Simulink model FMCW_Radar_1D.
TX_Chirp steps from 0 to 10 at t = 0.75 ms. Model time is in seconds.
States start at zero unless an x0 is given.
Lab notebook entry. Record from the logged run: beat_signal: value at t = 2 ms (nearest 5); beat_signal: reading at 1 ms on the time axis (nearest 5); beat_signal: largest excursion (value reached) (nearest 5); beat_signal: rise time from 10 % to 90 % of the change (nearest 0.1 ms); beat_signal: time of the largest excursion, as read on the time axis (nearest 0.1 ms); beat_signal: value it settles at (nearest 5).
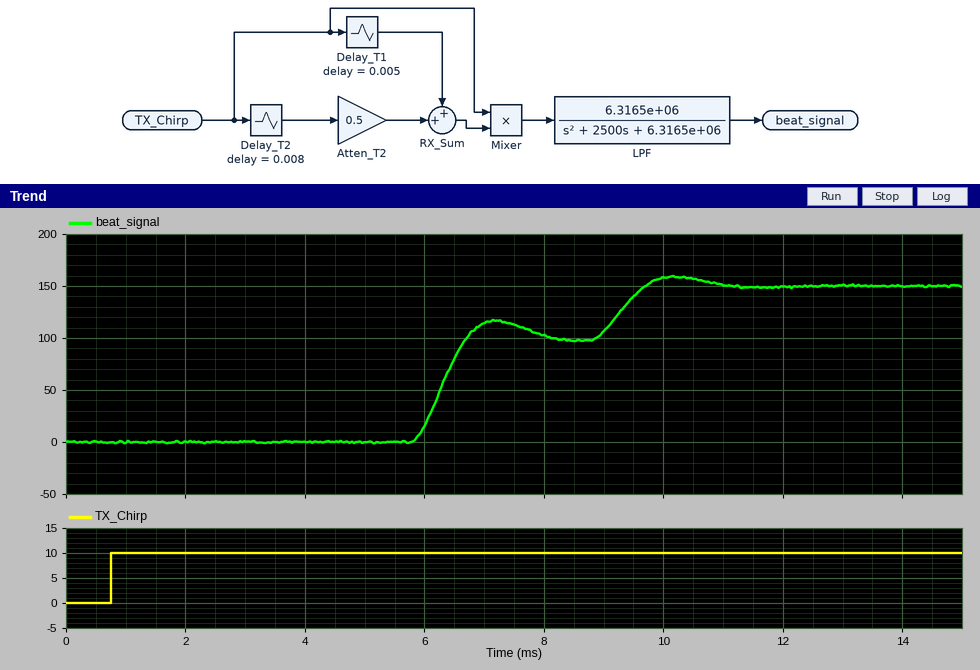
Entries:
0
0
160
3.4 ms
10.2 ms
150
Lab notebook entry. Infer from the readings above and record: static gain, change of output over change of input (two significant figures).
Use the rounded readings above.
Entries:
15
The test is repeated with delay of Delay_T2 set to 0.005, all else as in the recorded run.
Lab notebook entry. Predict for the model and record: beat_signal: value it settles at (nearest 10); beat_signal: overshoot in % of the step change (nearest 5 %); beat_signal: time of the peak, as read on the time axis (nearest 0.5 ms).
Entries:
150
15 %
7.0 ms
